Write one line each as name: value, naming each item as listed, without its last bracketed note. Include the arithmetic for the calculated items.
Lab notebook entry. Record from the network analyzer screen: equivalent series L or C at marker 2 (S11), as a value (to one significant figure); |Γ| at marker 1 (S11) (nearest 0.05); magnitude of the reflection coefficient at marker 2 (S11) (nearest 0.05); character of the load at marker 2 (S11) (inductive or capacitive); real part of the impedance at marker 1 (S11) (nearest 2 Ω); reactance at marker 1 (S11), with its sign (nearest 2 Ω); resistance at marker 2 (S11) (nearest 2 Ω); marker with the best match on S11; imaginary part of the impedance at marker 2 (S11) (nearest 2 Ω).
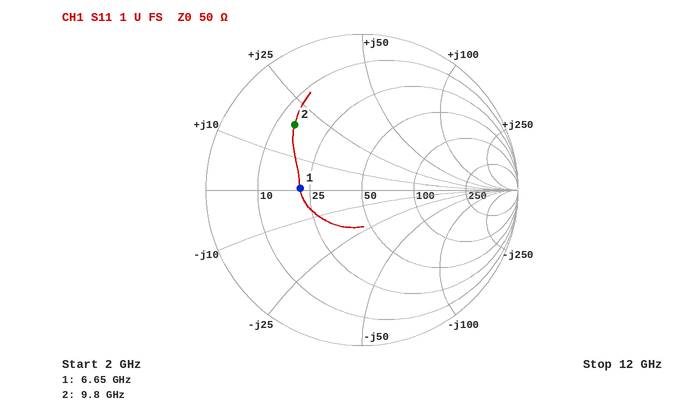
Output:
equivalent series L or C at marker 2 (S11), as a value: L = 18 Ω/(2π × 9.8 GHz) ≈ 292 pH, so 300 pH to one significant figure
|Γ| at marker 1 (S11): 0.40
magnitude of the reflection coefficient at marker 2 (S11): 0.60
character of the load at marker 2 (S11): inductive
real part of the impedance at marker 1 (S11): 22 Ω
reactance at marker 1 (S11), with its sign: 0 Ω
resistance at marker 2 (S11): 14 Ω
marker with the best match on S11: marker 1
imaginary part of the impedance at marker 2 (S11): +18 Ω
